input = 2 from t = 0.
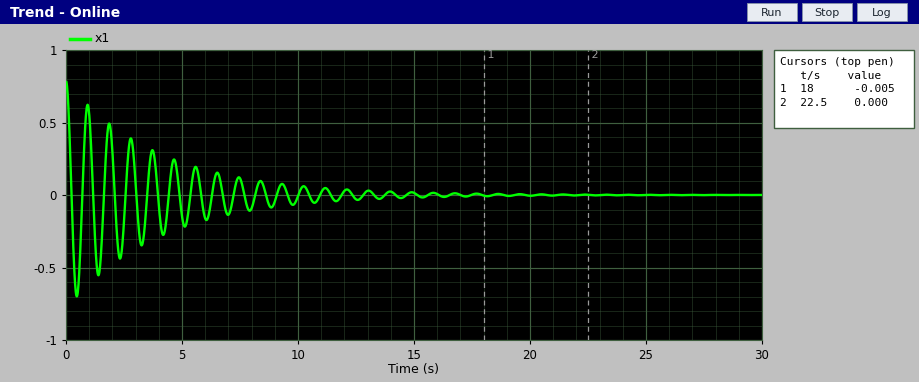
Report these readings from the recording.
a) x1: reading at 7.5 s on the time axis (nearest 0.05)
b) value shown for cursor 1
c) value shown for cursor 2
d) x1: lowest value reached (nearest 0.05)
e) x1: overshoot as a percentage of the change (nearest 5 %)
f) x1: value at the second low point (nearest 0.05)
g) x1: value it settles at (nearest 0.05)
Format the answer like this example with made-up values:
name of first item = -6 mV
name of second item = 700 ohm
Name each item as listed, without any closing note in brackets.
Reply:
x1: reading at 7.5 s on the time axis = 0.10
value shown for cursor 1 = -0.005
value shown for cursor 2 = 0.000
x1: lowest value reached = -0.70
x1: overshoot as a percentage of the change = 90 %
x1: value at the second low point = -0.55
x1: value it settles at = 0.00
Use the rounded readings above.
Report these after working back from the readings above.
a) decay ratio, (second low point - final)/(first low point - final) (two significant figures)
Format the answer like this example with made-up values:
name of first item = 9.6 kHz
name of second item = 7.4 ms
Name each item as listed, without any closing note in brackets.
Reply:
decay ratio, (second low point - final)/(first low point - final) = 0.79
